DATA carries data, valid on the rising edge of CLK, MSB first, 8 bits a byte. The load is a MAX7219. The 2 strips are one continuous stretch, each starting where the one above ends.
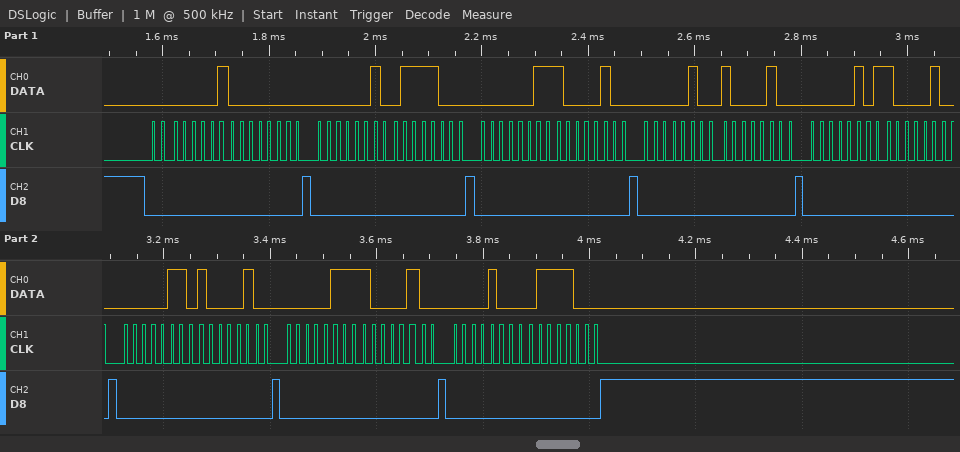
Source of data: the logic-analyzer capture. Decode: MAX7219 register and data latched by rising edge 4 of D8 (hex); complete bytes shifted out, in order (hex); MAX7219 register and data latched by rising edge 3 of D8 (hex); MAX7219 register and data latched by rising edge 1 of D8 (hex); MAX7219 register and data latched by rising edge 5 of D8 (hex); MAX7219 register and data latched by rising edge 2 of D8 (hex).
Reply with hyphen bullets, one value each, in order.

- register 0x4, data 0x84
- 01 00 02 78 03 84 04 84 05 84 06 84 07 84 08 78
- register 0x3, data 0x84
- register 0x1, data 0x00
- register 0x5, data 0x84
- register 0x2, data 0x78
